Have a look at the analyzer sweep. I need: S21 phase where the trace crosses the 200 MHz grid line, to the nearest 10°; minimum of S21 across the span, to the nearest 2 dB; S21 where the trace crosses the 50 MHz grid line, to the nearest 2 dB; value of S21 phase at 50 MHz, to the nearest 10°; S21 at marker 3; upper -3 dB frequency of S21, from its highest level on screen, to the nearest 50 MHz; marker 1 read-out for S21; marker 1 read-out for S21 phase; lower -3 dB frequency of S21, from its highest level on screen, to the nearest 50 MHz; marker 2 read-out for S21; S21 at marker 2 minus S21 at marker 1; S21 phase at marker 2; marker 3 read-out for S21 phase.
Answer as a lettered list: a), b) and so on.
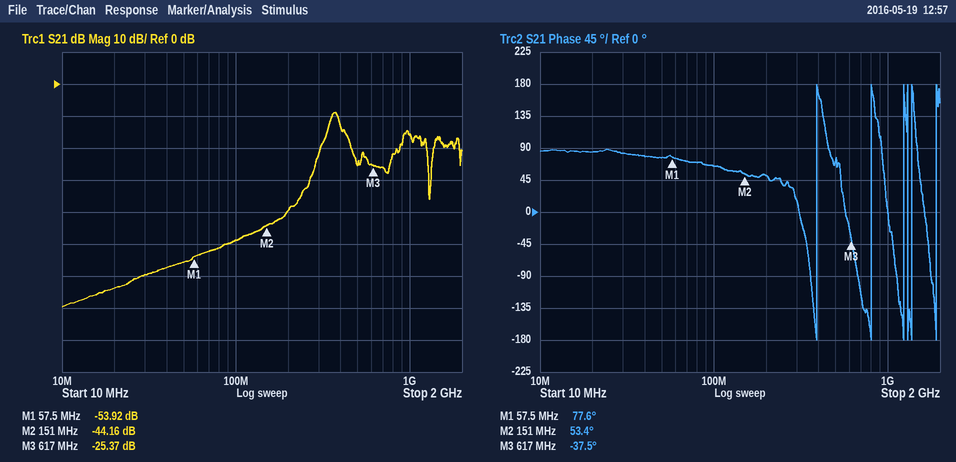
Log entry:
a) 50°
b) -70 dB
c) -56 dB
d) 80°
e) -25.37 dB
f) 400 MHz
g) -53.92 dB
h) 77.6°
i) 350 MHz
j) -44.16 dB
k) 9.76 dB
l) 53.4°
m) -37.5°
